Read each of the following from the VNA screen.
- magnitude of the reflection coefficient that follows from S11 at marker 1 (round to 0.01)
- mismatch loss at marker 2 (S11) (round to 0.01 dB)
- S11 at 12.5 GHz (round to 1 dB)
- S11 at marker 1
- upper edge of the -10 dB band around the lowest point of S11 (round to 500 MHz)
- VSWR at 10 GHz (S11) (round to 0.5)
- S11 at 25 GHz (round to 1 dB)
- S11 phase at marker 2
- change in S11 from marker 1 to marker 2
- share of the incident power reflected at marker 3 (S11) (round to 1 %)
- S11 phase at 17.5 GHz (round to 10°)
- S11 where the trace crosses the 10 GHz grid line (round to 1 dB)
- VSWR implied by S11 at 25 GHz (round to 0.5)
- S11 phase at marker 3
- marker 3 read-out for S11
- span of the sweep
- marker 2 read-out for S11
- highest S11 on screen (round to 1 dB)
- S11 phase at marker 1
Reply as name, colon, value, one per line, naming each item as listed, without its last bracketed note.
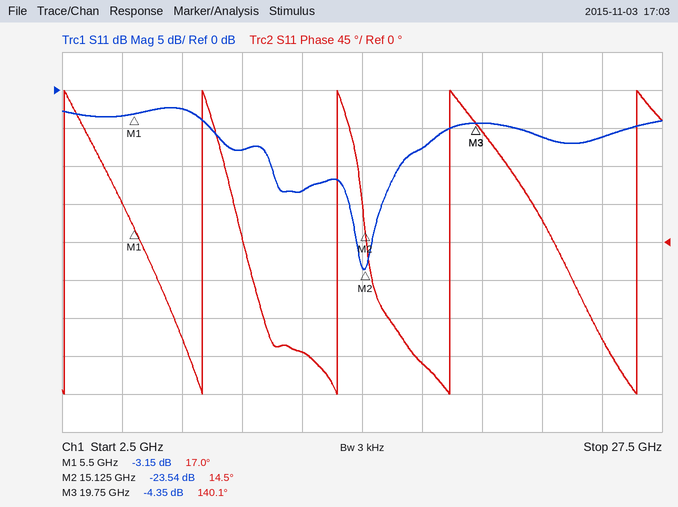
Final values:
magnitude of the reflection coefficient that follows from S11 at marker 1: 0.70
mismatch loss at marker 2 (S11): 0.02 dB
S11 at 12.5 GHz: -13 dB
S11 at marker 1: -3.15 dB
upper edge of the -10 dB band around the lowest point of S11: 16.5 GHz
VSWR at 10 GHz (S11): 2.5
S11 at 25 GHz: -6 dB
S11 phase at marker 2: 14.5°
change in S11 from marker 1 to marker 2: -20.39 dB
share of the incident power reflected at marker 3 (S11): 37 %
S11 phase at 17.5 GHz: -140°
S11 where the trace crosses the 10 GHz grid line: -8 dB
VSWR implied by S11 at 25 GHz: 3.0
S11 phase at marker 3: 140.1°
marker 3 read-out for S11: -4.35 dB
span of the sweep: 25 GHz
marker 2 read-out for S11: -23.54 dB
highest S11 on screen: -2 dB
S11 phase at marker 1: 17.0°
